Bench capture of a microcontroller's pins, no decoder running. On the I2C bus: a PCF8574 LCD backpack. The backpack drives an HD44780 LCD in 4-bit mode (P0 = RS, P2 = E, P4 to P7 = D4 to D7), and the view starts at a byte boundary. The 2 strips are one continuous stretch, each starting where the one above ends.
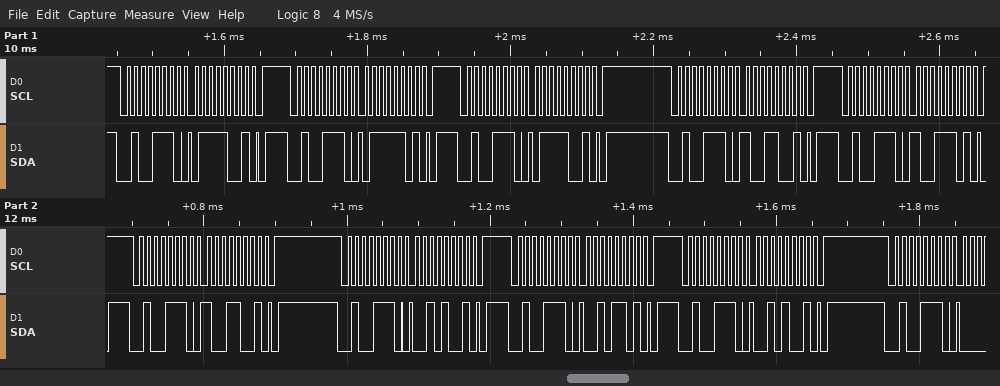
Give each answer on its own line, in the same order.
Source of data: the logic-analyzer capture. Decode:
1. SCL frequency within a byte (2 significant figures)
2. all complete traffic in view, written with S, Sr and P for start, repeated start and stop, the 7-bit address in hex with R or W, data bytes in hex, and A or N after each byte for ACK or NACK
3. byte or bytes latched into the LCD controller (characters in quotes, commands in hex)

100 kHz
S 27W A 79 A P S 27W A 7D A P S 27W A 79 A P S 27W A 99 A P S 27W A 9D A P S 27W A 99 A P S 27W A 29 A P S 27W A 2D A P S 27W A 29 A P S 27W A
'y'
